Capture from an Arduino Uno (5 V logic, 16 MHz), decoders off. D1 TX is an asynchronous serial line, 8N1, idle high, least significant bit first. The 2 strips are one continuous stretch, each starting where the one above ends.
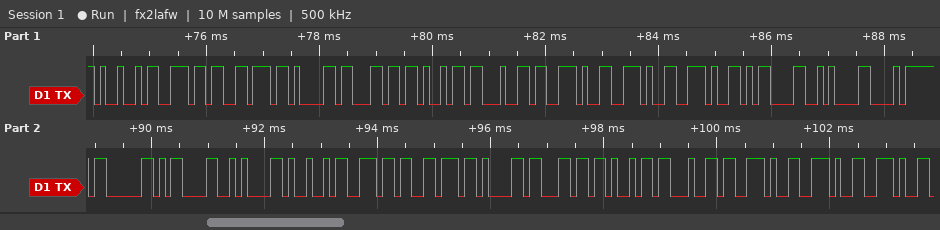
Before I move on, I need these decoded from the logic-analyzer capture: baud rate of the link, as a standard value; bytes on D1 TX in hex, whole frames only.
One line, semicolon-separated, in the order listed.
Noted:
9600 baud; 49 6E 76 61 6C 69 64 2E 2E 2E 0D 0A E8 03 0D 0A 49 6E 76 61 6C 69 64 2E 2E 2E
